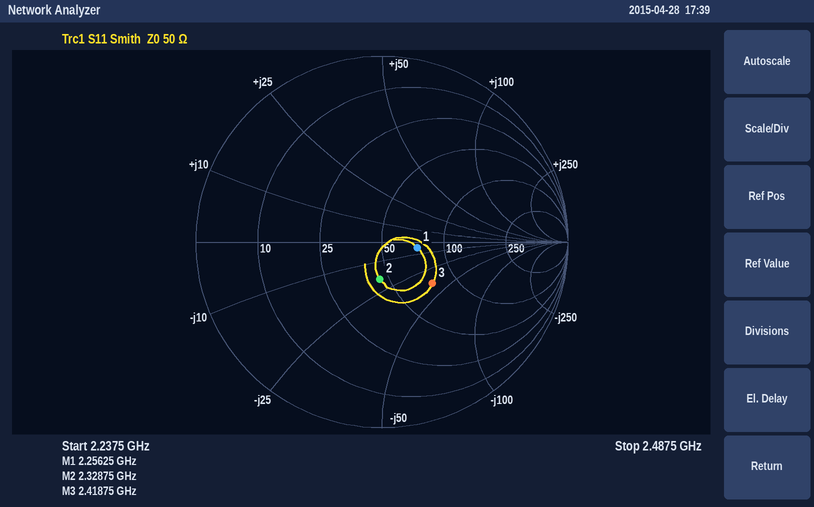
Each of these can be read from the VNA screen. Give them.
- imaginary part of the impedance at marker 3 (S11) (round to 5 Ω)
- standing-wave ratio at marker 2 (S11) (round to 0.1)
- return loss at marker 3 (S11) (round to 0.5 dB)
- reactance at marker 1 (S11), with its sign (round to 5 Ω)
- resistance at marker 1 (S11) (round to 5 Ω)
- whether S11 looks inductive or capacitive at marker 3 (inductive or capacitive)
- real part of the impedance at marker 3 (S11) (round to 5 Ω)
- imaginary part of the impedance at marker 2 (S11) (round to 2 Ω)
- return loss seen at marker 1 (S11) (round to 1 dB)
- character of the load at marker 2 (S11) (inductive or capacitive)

-40 Ω
1.5
9.0 dB
-5 Ω
75 Ω
capacitive
75 Ω
-18 Ω
14 dB
capacitive
